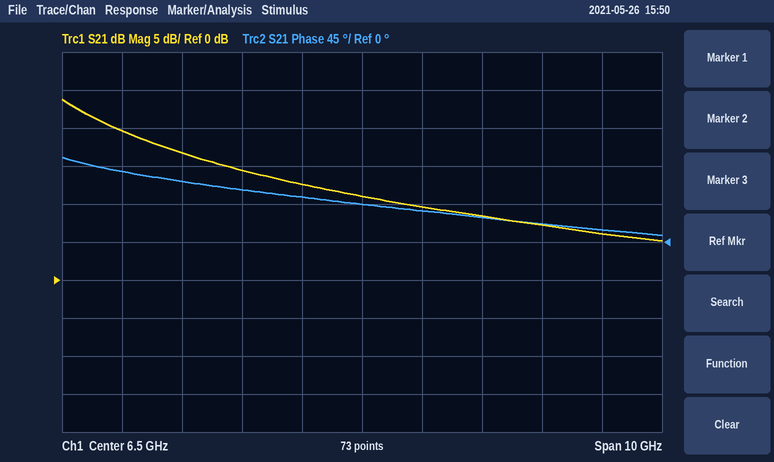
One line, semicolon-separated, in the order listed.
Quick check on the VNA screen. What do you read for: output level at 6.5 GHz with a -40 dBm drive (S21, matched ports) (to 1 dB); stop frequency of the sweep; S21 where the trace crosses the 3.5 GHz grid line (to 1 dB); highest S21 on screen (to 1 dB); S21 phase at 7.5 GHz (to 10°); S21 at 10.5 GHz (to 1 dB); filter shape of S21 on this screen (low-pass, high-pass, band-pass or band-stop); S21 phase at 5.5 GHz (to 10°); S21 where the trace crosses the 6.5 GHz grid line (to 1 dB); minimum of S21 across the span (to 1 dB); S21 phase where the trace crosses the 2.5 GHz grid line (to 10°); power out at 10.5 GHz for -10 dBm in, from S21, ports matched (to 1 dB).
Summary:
-29 dBm; 11.5 GHz; 17 dB; 24 dB; 40°; 6 dB; low-pass; 50°; 11 dB; 5 dB; 80°; -4 dBm
